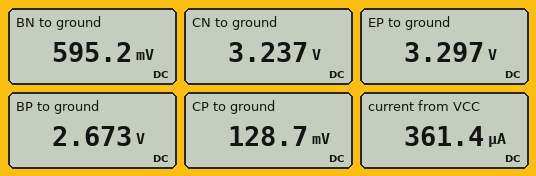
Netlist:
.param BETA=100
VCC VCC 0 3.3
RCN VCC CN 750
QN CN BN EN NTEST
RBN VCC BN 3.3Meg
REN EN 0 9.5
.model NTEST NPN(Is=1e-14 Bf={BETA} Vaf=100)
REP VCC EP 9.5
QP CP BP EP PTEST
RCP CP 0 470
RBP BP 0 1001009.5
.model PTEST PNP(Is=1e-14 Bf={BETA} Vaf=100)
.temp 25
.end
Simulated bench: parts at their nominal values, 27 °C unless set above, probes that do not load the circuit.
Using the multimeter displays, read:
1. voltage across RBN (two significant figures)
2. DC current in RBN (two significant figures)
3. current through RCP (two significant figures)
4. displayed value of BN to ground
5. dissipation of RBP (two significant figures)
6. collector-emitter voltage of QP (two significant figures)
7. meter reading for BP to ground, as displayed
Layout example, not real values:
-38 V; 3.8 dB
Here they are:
2.7 V; 820 nA; 270 µA; 595.2 mV; 7.1 µW; -3.2 V; 2.673 V
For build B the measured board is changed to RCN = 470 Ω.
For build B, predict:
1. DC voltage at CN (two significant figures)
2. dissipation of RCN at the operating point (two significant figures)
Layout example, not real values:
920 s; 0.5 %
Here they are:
3.3 V; 3.3 µW
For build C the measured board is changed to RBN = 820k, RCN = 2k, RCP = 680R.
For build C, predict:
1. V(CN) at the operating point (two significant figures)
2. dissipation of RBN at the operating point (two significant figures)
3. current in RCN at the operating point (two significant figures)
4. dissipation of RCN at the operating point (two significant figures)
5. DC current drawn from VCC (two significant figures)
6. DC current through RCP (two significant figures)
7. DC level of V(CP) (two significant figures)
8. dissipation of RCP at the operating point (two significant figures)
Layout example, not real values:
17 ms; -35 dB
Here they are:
2.6 V; 8.7 µW; 330 µA; 220 µW; 610 µA; 270 µA; 190 mV; 51 µW
